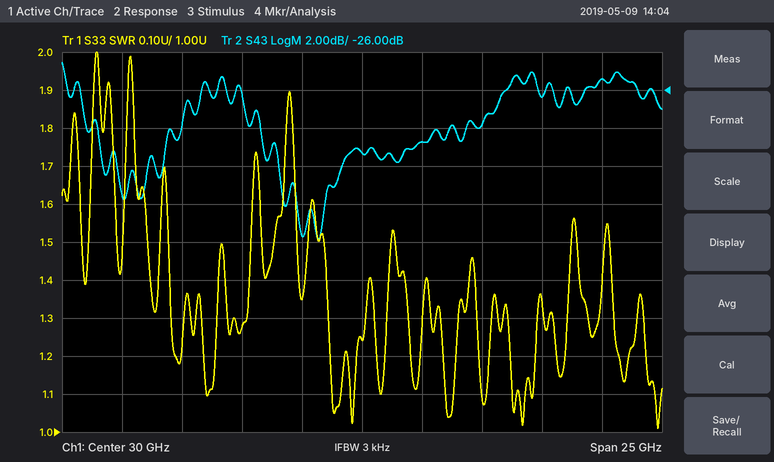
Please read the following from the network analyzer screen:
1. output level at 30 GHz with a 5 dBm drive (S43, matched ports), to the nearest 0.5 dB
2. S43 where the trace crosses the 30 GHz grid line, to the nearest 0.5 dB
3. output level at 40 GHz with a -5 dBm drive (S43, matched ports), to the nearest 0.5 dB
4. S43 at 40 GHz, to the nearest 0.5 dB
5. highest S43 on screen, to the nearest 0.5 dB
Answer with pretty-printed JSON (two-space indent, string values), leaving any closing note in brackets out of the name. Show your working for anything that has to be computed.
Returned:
{
  "output level at 30 GHz with a 5 dBm drive (S43, matched ports), to the nearest 0.5 dB": "5 dBm + (-29.5 dB) = -24.5 dBm",
  "S43 where the trace crosses the 30 GHz grid line, to the nearest 0.5 dB": "-29.5 dB",
  "output level at 40 GHz with a -5 dBm drive (S43, matched ports), to the nearest 0.5 dB": "-5 dBm + (-25.5 dB) = -30.5 dBm",
  "S43 at 40 GHz, to the nearest 0.5 dB": "-25.5 dB",
  "highest S43 on screen, to the nearest 0.5 dB": "-24.5 dB"
}
